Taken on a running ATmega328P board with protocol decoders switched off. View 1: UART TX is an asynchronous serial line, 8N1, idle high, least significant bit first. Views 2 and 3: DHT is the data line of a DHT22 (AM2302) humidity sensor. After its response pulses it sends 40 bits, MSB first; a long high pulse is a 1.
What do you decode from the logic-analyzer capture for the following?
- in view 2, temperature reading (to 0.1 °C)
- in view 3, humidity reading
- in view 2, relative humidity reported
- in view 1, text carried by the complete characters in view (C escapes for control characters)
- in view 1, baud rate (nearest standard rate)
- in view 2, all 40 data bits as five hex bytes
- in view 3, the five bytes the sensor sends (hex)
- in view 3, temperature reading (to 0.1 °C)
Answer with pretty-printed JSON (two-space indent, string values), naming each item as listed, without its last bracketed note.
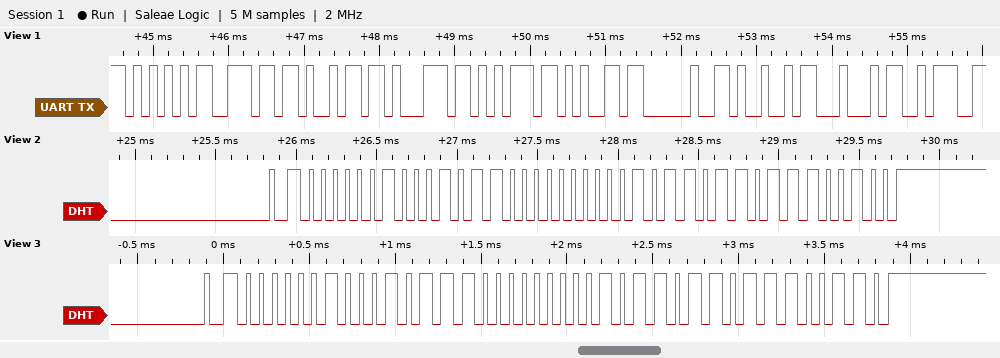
{
  "in view 2, temperature reading": "18.2 °C",
  "in view 3, humidity reading": "55.8 %",
  "in view 2, relative humidity reported": "55.6 %",
  "in view 1, text carried by the complete characters in view": "\"Unique ID:\"",
  "in view 1, baud rate": "9600 baud",
  "in view 2, all 40 data bits as five hex bytes": "02 2C 00 B6 E4",
  "in view 3, the five bytes the sensor sends": "02 2E 00 B6 E6",
  "in view 3, temperature reading": "18.2 °C"
}
